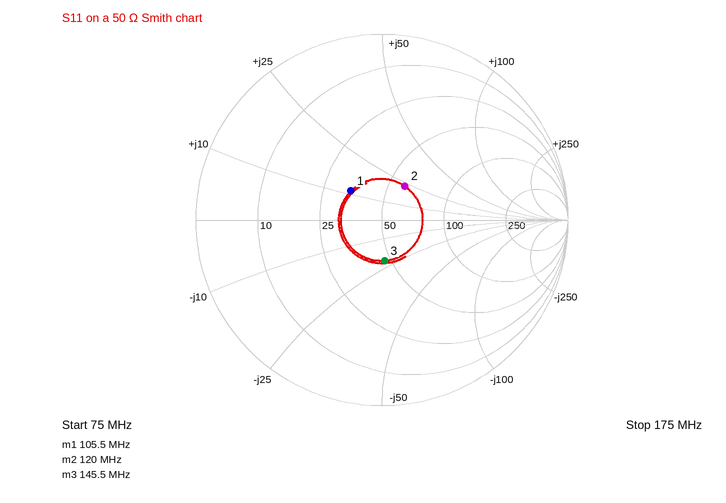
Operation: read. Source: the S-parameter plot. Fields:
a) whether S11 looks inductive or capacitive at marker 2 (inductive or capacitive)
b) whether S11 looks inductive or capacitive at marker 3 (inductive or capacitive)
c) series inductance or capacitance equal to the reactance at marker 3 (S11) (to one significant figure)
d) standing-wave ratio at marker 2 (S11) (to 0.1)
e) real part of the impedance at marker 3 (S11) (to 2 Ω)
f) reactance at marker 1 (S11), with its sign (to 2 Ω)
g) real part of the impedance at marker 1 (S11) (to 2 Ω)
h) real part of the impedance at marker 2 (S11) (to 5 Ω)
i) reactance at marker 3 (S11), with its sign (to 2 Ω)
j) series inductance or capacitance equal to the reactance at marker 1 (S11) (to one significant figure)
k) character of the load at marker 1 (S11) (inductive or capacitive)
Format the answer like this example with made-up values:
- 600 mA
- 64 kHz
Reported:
- inductive
- capacitive
- 50 pF
- 1.6
- 46 Ω
- +12 Ω
- 34 Ω
- 60 Ω
- -22 Ω
- 20 nH
- inductive
